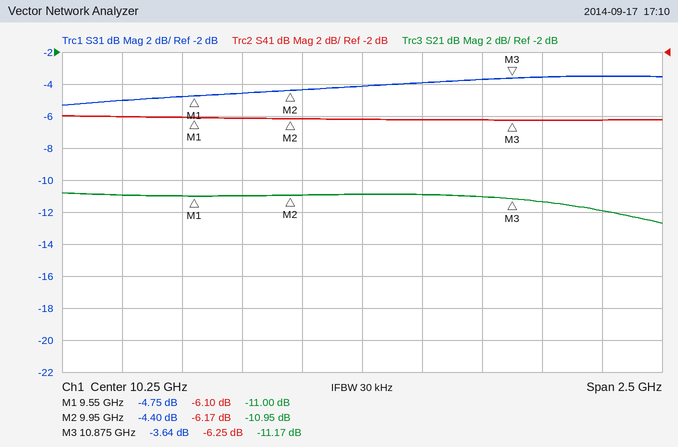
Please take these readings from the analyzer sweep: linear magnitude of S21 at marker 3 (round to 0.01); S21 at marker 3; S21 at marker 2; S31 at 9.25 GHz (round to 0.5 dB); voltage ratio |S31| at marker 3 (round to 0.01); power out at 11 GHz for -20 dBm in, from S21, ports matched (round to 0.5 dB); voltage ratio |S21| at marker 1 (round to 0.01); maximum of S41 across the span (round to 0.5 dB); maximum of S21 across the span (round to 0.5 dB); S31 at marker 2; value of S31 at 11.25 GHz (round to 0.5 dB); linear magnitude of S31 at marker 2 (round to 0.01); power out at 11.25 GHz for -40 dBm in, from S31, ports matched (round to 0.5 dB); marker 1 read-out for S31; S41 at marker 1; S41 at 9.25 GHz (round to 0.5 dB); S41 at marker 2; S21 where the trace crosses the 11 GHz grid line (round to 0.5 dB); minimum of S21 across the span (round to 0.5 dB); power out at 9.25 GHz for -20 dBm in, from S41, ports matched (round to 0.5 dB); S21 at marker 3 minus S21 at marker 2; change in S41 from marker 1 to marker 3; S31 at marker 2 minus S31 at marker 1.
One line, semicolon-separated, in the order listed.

0.28; -11.17 dB; -10.95 dB; -5.0 dB; 0.66; -31.5 dBm; 0.28; -6.0 dB; -11.0 dB; -4.40 dB; -3.5 dB; 0.60; -43.5 dBm; -4.75 dB; -6.10 dB; -6.0 dB; -6.17 dB; -11.5 dB; -12.5 dB; -26.0 dBm; -0.22 dB; -0.15 dB; 0.35 dB
